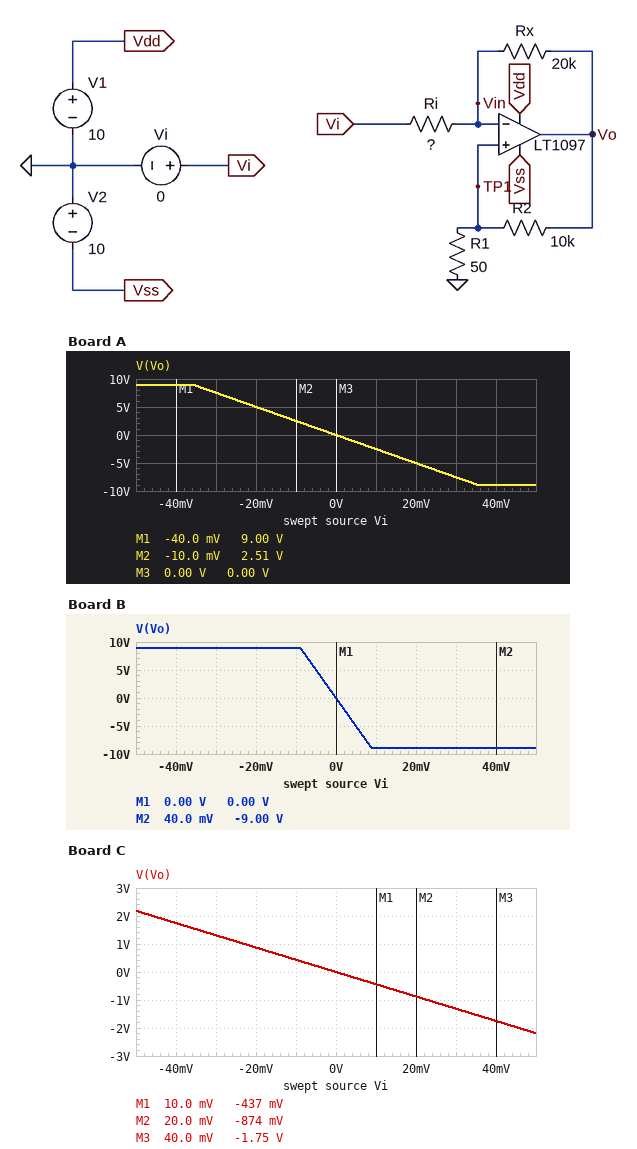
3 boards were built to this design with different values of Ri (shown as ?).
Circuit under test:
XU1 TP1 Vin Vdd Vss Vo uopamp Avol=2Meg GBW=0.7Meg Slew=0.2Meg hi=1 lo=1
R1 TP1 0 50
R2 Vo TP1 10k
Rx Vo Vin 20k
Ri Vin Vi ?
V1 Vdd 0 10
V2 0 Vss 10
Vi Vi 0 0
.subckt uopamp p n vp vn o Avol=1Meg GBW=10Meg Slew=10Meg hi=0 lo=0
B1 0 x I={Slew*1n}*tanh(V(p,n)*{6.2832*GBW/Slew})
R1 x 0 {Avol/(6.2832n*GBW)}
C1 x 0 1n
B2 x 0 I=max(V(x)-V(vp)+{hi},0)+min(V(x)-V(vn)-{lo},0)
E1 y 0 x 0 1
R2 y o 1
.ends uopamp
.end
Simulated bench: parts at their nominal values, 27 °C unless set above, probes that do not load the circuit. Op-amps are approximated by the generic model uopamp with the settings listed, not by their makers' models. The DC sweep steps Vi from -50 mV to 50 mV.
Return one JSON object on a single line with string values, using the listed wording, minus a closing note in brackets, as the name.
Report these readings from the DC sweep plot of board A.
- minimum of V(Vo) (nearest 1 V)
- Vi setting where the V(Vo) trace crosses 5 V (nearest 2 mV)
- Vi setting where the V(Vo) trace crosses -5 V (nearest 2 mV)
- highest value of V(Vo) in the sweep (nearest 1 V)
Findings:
{"minimum of V(Vo)": "-9 V", "Vi setting where the V(Vo) trace crosses 5 V": "-20 mV", "Vi setting where the V(Vo) trace crosses -5 V": "20 mV", "highest value of V(Vo) in the sweep": "9 V"}
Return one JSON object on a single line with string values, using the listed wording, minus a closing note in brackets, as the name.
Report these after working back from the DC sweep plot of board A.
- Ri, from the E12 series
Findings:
{"Ri, from the E12 series": "180 Ω"}
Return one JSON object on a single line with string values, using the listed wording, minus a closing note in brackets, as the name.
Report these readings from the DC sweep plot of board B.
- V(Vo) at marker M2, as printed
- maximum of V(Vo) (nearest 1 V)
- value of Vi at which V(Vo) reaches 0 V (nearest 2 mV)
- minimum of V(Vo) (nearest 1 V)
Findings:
{"V(Vo) at marker M2, as printed": "-9.00 V", "maximum of V(Vo)": "9 V", "value of Vi at which V(Vo) reaches 0 V": "0 V", "minimum of V(Vo)": "-9 V"}
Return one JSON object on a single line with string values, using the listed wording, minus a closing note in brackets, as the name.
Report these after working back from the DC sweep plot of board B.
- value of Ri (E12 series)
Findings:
{"value of Ri": "120 Ω"}
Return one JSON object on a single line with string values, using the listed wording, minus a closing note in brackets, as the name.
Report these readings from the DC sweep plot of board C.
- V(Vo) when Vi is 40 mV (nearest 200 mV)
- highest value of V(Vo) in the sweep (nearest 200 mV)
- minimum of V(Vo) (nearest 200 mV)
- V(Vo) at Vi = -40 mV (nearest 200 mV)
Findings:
{"V(Vo) when Vi is 40 mV": "-1.8 V", "highest value of V(Vo) in the sweep": "2.2 V", "minimum of V(Vo)": "-2.2 V", "V(Vo) at Vi = -40 mV": "1.8 V"}
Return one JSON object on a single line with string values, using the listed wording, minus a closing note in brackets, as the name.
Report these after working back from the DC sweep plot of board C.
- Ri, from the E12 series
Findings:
{"Ri, from the E12 series": "560 Ω"}
